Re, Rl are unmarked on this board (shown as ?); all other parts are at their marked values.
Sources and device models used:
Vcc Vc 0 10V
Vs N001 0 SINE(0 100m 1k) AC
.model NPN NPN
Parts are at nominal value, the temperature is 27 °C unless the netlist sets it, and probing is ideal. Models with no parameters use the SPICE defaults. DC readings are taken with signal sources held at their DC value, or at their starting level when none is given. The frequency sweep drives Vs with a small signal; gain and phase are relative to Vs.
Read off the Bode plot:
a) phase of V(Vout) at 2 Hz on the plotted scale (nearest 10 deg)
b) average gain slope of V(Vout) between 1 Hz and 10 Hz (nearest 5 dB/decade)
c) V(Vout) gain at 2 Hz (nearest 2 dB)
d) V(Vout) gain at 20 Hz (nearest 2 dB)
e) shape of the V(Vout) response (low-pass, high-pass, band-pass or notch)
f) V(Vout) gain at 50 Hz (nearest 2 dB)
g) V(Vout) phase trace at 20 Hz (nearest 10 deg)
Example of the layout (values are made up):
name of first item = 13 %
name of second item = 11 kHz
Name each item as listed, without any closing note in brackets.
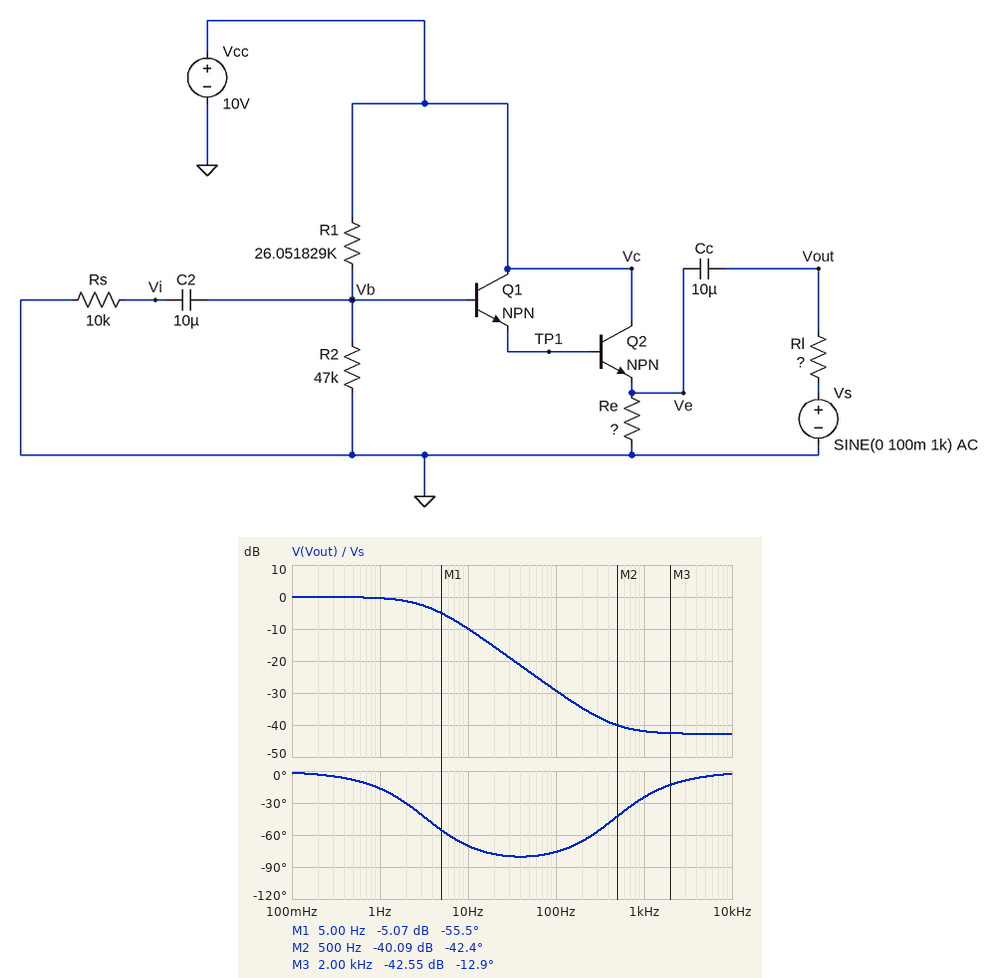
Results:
phase of V(Vout) at 2 Hz on the plotted scale = -30 deg
average gain slope of V(Vout) between 1 Hz and 10 Hz = -10 dB/decade
V(Vout) gain at 2 Hz = -2 dB
V(Vout) gain at 20 Hz = -16 dB
shape of the V(Vout) response = low-pass
V(Vout) gain at 50 Hz = -24 dB
V(Vout) phase trace at 20 Hz = -80 deg
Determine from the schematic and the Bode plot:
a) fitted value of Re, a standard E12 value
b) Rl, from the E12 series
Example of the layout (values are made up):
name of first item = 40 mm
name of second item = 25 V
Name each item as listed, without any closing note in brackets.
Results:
fitted value of Re, a standard E12 value = 3.3 kΩ
Rl, from the E12 series = 4.7 kΩ
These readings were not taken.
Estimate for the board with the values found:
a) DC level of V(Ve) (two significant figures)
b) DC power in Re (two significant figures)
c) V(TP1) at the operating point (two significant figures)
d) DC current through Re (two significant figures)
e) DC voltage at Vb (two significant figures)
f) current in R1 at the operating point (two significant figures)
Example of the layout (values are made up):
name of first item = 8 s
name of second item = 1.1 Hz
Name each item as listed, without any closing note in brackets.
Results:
DC level of V(Ve) = 5.0 V
DC power in Re = 7.5 mW
V(TP1) at the operating point = 5.8 V
DC current through Re = 1.5 mA
DC voltage at Vb = 6.4 V
current in R1 at the operating point = 140 µA
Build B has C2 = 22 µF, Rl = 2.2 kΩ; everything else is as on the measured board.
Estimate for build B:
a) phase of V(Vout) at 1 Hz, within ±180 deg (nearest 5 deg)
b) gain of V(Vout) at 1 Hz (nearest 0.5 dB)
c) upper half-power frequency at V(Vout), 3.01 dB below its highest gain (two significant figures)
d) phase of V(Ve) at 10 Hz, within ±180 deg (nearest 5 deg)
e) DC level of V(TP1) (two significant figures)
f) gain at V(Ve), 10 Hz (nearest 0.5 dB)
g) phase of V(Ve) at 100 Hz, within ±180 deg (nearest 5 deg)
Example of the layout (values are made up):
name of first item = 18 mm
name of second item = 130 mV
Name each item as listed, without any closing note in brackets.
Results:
phase of V(Vout) at 1 Hz, within ±180 deg = -10 deg
gain of V(Vout) at 1 Hz = 0 dB
upper half-power frequency at V(Vout), 3.01 dB below its highest gain = 7.1 Hz
phase of V(Ve) at 10 Hz, within ±180 deg = 35 deg
DC level of V(TP1) = 5.8 V
gain at V(Ve), 10 Hz = -38.0 dB
phase of V(Ve) at 100 Hz, within ±180 deg = 5 deg
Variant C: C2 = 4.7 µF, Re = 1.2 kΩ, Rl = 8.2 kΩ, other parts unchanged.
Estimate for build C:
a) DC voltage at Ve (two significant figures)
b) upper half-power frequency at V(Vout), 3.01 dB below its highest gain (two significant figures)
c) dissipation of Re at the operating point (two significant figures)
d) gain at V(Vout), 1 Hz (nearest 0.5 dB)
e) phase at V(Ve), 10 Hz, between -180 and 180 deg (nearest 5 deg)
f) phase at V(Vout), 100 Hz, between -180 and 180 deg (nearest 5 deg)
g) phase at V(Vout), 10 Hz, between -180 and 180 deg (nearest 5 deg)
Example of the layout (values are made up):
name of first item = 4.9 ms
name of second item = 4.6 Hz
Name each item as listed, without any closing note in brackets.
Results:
DC voltage at Ve = 4.9 V
upper half-power frequency at V(Vout), 3.01 dB below its highest gain = 1.9 Hz
dissipation of Re at the operating point = 20 mW
gain at V(Vout), 1 Hz = -1.0 dB
phase at V(Ve), 10 Hz, between -180 and 180 deg = 10 deg
phase at V(Vout), 100 Hz, between -180 and 180 deg = -85 deg
phase at V(Vout), 10 Hz, between -180 and 180 deg = -80 deg
